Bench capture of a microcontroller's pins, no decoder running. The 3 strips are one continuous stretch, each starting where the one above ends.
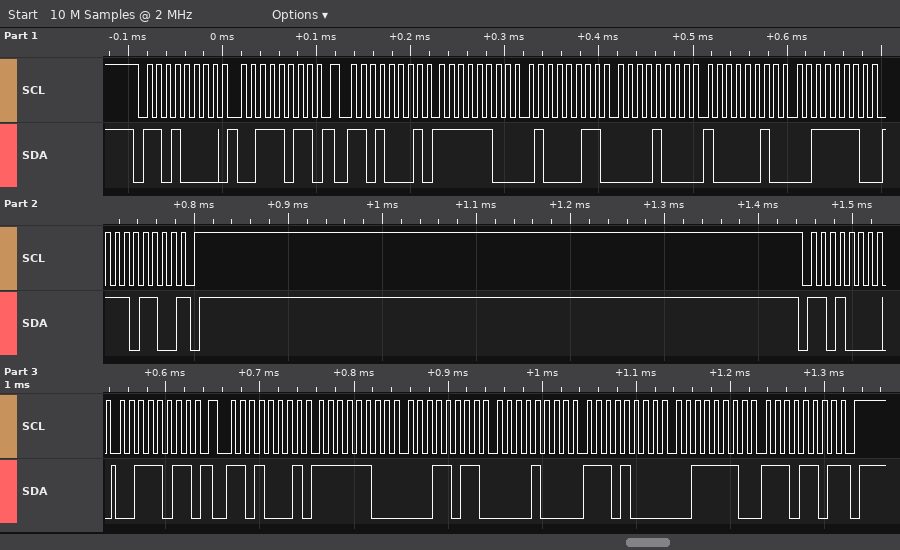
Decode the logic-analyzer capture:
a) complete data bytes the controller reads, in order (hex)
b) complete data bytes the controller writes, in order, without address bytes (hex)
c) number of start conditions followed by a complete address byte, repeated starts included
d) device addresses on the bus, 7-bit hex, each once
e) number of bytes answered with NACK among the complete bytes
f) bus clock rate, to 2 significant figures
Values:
FC 43 08 82 3E EC FC 1B 08 E8 3E ED
3B 3B
4
0x68
2
100 kHz
